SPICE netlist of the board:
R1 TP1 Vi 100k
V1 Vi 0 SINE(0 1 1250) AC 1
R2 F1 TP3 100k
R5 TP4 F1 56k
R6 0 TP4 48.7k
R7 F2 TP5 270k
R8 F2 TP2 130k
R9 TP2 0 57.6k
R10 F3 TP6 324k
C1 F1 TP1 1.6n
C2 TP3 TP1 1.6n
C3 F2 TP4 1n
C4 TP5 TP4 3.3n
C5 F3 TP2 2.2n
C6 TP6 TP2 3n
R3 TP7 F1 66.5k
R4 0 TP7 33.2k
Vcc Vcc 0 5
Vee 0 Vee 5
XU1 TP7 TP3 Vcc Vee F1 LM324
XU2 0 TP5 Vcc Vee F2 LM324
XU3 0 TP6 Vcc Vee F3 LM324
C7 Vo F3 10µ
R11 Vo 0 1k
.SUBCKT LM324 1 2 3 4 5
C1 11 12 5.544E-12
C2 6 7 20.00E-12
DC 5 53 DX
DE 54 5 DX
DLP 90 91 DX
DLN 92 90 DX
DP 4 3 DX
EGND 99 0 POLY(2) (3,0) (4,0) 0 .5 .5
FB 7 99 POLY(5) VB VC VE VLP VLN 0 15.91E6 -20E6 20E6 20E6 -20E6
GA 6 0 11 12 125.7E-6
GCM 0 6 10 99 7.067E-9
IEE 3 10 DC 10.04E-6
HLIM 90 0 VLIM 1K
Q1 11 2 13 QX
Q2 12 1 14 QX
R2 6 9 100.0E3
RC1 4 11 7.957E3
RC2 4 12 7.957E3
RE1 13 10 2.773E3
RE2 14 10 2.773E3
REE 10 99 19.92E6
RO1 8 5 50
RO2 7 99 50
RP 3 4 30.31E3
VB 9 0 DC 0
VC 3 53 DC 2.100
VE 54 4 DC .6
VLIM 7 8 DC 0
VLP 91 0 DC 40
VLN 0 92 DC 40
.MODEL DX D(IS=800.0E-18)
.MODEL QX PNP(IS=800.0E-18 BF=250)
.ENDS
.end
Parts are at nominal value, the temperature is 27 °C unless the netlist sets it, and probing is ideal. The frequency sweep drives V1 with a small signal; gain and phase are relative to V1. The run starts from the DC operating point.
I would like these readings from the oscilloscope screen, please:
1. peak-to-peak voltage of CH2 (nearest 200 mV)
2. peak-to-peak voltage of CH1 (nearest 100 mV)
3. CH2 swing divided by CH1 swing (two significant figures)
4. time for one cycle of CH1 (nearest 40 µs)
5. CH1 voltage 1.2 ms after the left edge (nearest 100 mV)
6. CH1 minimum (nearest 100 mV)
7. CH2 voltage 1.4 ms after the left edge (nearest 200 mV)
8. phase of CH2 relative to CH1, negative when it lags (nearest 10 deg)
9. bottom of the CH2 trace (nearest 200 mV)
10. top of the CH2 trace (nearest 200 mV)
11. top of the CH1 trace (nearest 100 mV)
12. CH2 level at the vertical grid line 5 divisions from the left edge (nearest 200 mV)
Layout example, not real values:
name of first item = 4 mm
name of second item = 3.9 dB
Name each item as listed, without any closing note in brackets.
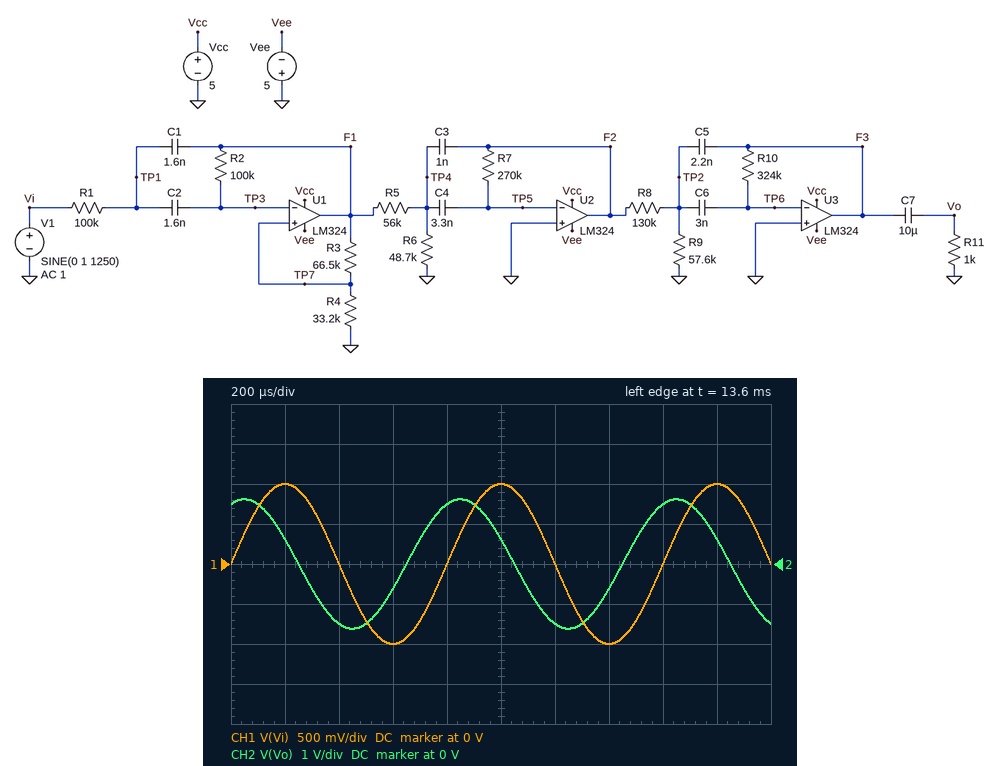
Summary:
peak-to-peak voltage of CH2 = 3.2 V
peak-to-peak voltage of CH1 = 2.0 V
CH2 swing divided by CH1 swing = 1.6
time for one cycle of CH1 = 800 µs
CH1 voltage 1.2 ms after the left edge = 0 V
CH1 minimum = -1.0 V
CH2 voltage 1.4 ms after the left edge = -600 mV
phase of CH2 relative to CH1, negative when it lags = 70 deg
bottom of the CH2 trace = -1.6 V
top of the CH2 trace = 1.6 V
top of the CH1 trace = 1.0 V
CH2 level at the vertical grid line 5 divisions from the left edge = 600 mV
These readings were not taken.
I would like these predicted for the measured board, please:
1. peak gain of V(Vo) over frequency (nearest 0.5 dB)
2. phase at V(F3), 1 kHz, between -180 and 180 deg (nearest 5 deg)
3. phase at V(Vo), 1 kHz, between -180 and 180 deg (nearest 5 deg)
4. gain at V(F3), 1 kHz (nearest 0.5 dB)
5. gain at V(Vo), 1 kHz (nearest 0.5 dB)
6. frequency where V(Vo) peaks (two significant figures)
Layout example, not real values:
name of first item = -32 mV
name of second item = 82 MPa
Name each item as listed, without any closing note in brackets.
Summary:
peak gain of V(Vo) over frequency = 9.0 dB
phase at V(F3), 1 kHz, between -180 and 180 deg = 125 deg
phase at V(Vo), 1 kHz, between -180 and 180 deg = 125 deg
gain at V(F3), 1 kHz = 8.0 dB
gain at V(Vo), 1 kHz = 8.0 dB
frequency where V(Vo) peaks = 840 Hz
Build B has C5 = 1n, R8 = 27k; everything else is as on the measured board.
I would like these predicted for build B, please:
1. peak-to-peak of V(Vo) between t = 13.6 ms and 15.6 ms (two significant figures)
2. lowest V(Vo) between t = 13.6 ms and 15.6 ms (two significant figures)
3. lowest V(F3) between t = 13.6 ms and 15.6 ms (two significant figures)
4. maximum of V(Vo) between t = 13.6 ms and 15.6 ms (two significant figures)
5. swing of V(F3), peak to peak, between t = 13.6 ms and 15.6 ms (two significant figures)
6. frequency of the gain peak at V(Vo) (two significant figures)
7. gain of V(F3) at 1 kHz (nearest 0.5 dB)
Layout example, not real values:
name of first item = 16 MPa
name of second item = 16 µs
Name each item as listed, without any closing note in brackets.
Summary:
peak-to-peak of V(Vo) between t = 13.6 ms and 15.6 ms = 8.6 V
lowest V(Vo) between t = 13.6 ms and 15.6 ms = -4.8 V
lowest V(F3) between t = 13.6 ms and 15.6 ms = -5.0 V
maximum of V(Vo) between t = 13.6 ms and 15.6 ms = 3.8 V
swing of V(F3), peak to peak, between t = 13.6 ms and 15.6 ms = 8.5 V
frequency of the gain peak at V(Vo) = 1.1 kHz
gain of V(F3) at 1 kHz = 29.0 dB
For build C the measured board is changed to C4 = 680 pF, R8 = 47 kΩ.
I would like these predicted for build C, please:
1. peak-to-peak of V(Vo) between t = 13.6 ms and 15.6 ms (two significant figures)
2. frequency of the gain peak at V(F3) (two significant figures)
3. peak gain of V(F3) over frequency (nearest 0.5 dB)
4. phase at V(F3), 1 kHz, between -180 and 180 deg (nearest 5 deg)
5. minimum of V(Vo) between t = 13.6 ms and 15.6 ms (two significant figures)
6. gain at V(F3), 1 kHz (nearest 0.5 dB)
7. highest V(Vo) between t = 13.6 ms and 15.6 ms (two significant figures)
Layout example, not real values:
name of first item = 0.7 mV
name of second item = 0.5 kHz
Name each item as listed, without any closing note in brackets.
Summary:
peak-to-peak of V(Vo) between t = 13.6 ms and 15.6 ms = 2.6 V
frequency of the gain peak at V(F3) = 800 Hz
peak gain of V(F3) over frequency = 4.0 dB
phase at V(F3), 1 kHz, between -180 and 180 deg = -165 deg
minimum of V(Vo) between t = 13.6 ms and 15.6 ms = -1.3 V
gain at V(F3), 1 kHz = 3.0 dB
highest V(Vo) between t = 13.6 ms and 15.6 ms = 1.3 V
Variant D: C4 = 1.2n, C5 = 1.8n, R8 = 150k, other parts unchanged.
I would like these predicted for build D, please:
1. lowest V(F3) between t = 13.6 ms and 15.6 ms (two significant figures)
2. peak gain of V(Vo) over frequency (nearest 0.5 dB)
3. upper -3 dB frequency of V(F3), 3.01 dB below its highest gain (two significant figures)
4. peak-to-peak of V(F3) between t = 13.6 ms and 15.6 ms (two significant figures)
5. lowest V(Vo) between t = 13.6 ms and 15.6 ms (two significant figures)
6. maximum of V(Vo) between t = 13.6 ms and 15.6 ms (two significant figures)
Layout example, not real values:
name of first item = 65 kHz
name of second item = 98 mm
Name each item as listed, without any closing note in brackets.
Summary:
lowest V(F3) between t = 13.6 ms and 15.6 ms = -960 mV
peak gain of V(Vo) over frequency = -0.5 dB
upper -3 dB frequency of V(F3), 3.01 dB below its highest gain = 1.8 kHz
peak-to-peak of V(F3) between t = 13.6 ms and 15.6 ms = 1.9 V
lowest V(Vo) between t = 13.6 ms and 15.6 ms = -950 mV
maximum of V(Vo) between t = 13.6 ms and 15.6 ms = 950 mV
